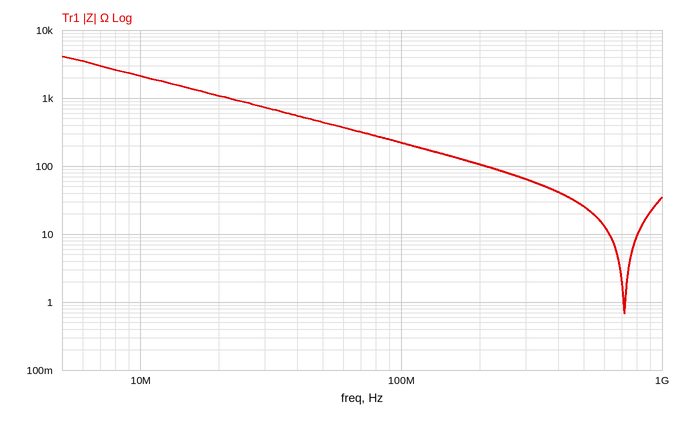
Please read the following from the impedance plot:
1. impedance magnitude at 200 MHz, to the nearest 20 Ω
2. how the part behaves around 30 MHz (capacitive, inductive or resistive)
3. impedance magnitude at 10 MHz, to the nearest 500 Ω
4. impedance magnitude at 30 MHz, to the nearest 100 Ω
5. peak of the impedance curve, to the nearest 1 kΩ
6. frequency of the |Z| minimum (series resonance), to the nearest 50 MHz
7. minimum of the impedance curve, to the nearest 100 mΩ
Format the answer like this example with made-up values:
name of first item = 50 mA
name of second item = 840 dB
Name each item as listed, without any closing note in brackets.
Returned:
impedance magnitude at 200 MHz, to the nearest 20 Ω = 100 Ω
how the part behaves around 30 MHz = capacitive
impedance magnitude at 10 MHz, to the nearest 500 Ω = 2.0 kΩ
impedance magnitude at 30 MHz, to the nearest 100 Ω = 700 Ω
peak of the impedance curve, to the nearest 1 kΩ = 4 kΩ
frequency of the |Z| minimum (series resonance), to the nearest 50 MHz = 700 MHz
minimum of the impedance curve, to the nearest 100 mΩ = 700 mΩ
